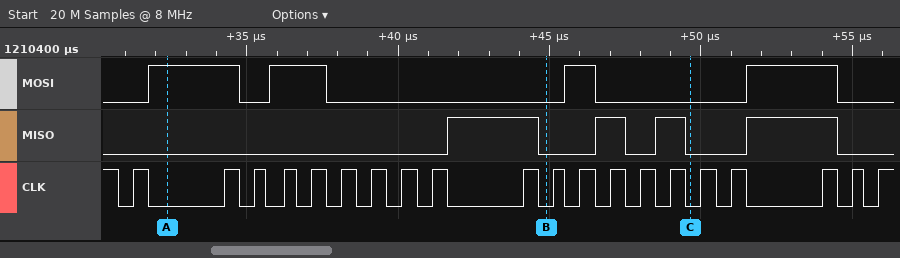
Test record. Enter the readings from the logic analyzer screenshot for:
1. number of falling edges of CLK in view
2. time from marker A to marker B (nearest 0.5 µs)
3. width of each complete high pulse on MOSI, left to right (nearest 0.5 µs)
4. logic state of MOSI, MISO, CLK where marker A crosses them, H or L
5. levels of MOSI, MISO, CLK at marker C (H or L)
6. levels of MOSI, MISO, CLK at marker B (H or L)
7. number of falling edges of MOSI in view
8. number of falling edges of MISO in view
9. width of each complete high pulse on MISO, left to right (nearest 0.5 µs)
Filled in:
20
12.5 µs
3 µs, 2 µs, 1 µs, 3 µs
MOSI=H, MISO=L, CLK=L
MOSI=L, MISO=L, CLK=L
MOSI=L, MISO=L, CLK=L
4
4
3 µs, 1 µs, 1 µs, 3 µs
